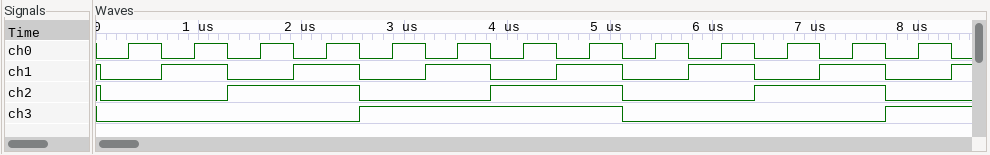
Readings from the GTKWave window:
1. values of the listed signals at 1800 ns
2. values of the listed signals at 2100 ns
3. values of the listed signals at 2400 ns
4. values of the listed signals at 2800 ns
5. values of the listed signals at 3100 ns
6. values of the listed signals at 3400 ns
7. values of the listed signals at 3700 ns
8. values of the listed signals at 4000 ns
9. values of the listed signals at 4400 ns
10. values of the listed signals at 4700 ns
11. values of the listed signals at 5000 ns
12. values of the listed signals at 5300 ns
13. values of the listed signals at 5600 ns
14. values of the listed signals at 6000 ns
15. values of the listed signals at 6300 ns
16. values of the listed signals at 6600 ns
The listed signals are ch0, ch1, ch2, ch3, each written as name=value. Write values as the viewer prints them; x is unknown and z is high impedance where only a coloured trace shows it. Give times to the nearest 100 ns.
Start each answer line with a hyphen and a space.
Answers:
- ch0=1, ch1=0, ch2=1, ch3=0
- ch0=0, ch1=1, ch2=1, ch3=0
- ch0=1, ch1=1, ch2=1, ch3=0
- ch0=0, ch1=0, ch2=0, ch3=1
- ch0=1, ch1=0, ch2=0, ch3=1
- ch0=0, ch1=1, ch2=0, ch3=1
- ch0=1, ch1=1, ch2=0, ch3=1
- ch0=0, ch1=0, ch2=1, ch3=1
- ch0=1, ch1=0, ch2=1, ch3=1
- ch0=0, ch1=1, ch2=1, ch3=1
- ch0=1, ch1=1, ch2=1, ch3=1
- ch0=0, ch1=0, ch2=0, ch3=0
- ch0=1, ch1=0, ch2=0, ch3=0
- ch0=0, ch1=1, ch2=0, ch3=0
- ch0=1, ch1=1, ch2=0, ch3=0
- ch0=0, ch1=0, ch2=1, ch3=0
